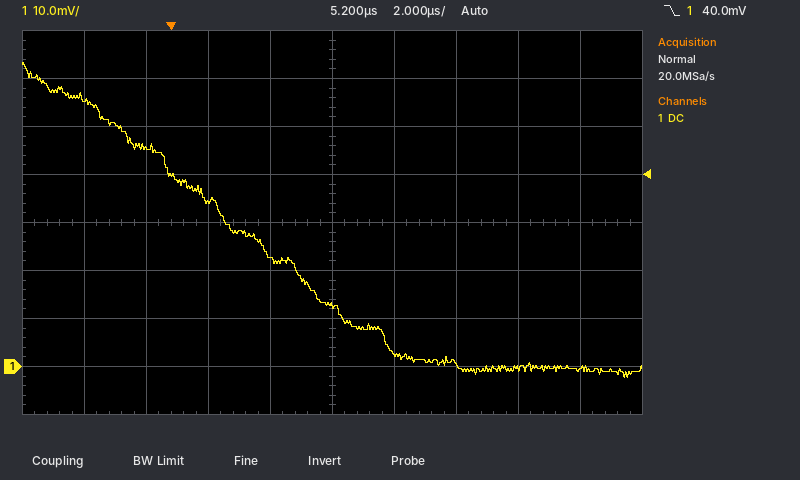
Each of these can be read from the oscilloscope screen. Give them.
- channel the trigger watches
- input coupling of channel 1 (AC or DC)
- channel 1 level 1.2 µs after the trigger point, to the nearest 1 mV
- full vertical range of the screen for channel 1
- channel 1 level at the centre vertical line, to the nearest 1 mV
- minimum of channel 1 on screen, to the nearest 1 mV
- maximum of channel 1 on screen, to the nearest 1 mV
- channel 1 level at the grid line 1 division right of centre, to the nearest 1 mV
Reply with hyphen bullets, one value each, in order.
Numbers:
- channel 1
- DC
- 34 mV
- 80 mV
- 13 mV
- -2 mV
- 63 mV
- 3 mV
